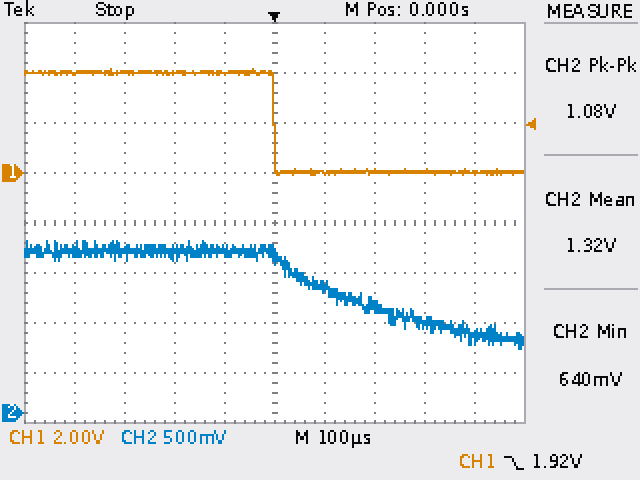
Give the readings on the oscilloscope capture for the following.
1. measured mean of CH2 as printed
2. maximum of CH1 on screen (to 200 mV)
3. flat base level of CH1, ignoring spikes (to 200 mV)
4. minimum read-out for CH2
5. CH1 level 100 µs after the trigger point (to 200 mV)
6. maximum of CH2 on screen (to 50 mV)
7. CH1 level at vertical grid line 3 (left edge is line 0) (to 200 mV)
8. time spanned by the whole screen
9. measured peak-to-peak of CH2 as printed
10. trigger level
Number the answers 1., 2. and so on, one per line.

1. 1.32 V
2. 4.2 V
3. 0.0 V
4. 640 mV
5. 0.0 V
6. 1.70 V
7. 4.0 V
8. 1 ms
9. 1.08 V
10. 1.92 V
